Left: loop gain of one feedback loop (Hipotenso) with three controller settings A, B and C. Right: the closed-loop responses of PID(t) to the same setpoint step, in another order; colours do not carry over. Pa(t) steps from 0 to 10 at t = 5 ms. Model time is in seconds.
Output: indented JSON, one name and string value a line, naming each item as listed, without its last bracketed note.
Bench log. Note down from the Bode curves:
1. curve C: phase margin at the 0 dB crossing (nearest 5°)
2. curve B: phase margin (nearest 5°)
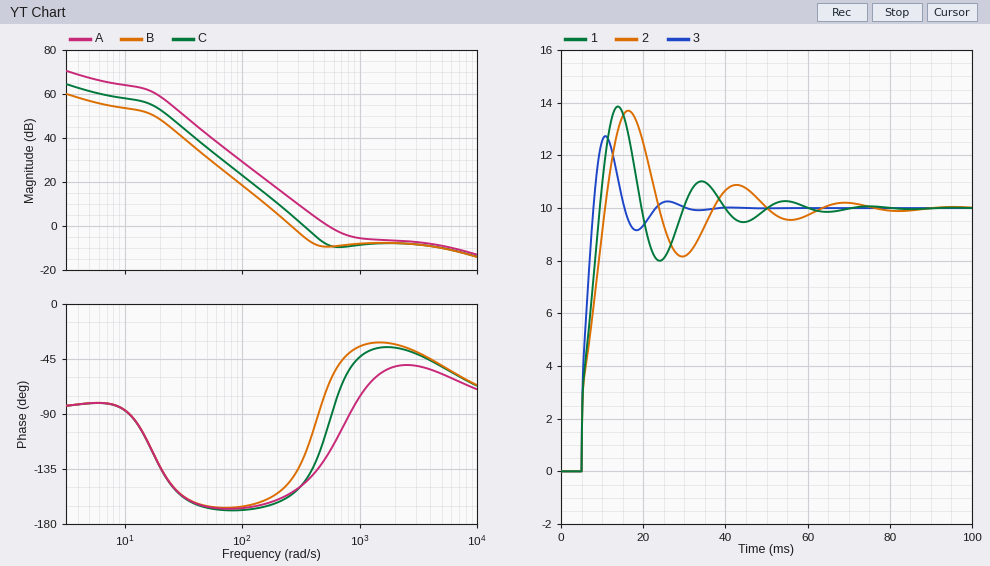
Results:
{
  "curve C: phase margin at the 0 dB crossing": "35°",
  "curve B: phase margin": "35°"
}
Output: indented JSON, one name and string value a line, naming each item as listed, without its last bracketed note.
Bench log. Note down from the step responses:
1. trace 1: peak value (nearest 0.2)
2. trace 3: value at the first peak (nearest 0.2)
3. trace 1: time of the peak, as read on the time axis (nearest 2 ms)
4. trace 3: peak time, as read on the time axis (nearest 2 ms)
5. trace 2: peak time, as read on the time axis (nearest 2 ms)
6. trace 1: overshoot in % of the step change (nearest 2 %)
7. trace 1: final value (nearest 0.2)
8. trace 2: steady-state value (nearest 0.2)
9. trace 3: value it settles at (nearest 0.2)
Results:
{
  "trace 1: peak value": "13.8",
  "trace 3: value at the first peak": "12.8",
  "trace 1: time of the peak, as read on the time axis": "14 ms",
  "trace 3: peak time, as read on the time axis": "10 ms",
  "trace 2: peak time, as read on the time axis": "16 ms",
  "trace 1: overshoot in % of the step change": "38 %",
  "trace 1: final value": "10.0",
  "trace 2: steady-state value": "10.0",
  "trace 3: value it settles at": "10.0"
}
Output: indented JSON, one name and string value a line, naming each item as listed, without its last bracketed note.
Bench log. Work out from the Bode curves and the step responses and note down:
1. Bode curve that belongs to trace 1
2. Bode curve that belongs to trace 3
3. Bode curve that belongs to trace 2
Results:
{
  "Bode curve that belongs to trace 1": "C",
  "Bode curve that belongs to trace 3": "A",
  "Bode curve that belongs to trace 2": "B"
}
